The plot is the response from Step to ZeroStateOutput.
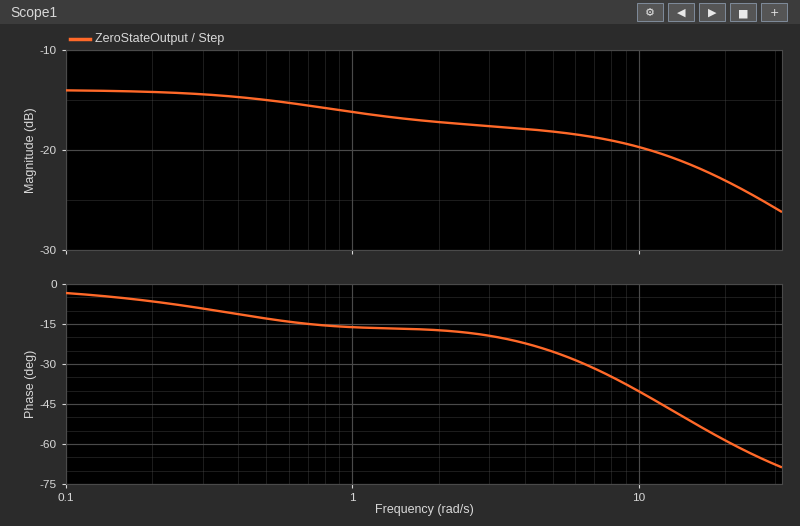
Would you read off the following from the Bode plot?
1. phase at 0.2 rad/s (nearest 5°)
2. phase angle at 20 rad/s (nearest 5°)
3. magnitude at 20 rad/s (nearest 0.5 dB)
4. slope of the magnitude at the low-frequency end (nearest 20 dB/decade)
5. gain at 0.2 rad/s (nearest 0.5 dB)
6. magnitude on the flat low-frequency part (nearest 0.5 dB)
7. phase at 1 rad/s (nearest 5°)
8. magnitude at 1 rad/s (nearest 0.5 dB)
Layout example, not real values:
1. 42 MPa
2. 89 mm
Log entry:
1. -5°
2. -60°
3. -23.0 dB
4. 0 dB/decade
5. -14.0 dB
6. -14.0 dB
7. -15°
8. -16.0 dB
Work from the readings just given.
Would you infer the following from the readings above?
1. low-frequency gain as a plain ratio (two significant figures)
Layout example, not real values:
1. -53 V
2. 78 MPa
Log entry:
1. 0.20
